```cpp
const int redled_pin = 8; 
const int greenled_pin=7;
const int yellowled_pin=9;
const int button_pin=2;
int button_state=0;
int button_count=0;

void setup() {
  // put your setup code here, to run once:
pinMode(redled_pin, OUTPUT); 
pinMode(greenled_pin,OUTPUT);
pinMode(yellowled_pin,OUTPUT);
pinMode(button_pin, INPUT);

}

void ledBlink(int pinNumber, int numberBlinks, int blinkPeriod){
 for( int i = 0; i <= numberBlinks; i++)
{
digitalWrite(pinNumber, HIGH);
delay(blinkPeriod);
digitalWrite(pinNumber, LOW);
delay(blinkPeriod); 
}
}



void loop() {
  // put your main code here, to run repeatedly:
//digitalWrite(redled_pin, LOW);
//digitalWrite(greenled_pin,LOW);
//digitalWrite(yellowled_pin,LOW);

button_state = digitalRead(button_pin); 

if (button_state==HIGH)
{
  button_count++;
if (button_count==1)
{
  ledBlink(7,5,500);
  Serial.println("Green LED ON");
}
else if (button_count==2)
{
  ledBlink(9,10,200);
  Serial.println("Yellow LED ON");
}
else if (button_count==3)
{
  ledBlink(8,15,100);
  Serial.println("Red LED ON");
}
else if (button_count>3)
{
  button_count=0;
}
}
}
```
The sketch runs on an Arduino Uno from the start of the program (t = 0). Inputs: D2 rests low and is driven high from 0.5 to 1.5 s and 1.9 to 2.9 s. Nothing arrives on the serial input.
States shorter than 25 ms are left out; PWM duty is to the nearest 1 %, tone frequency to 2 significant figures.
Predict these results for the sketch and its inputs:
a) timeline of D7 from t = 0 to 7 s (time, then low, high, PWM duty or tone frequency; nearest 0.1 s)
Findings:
0 s low; 0.5 s high; 1 s low; 1.5 s high; 2 s low; 2.5 s high; 3 s low; 3.5 s high; 4 s low; 4.5 s high; 5 s low; 5.5 s high; 6 s low
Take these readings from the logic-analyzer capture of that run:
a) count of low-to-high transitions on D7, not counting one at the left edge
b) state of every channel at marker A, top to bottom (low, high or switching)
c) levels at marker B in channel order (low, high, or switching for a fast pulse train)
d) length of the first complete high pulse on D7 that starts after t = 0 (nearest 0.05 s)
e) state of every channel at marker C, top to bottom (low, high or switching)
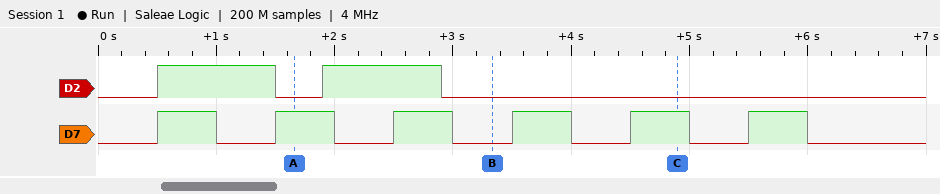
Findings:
6
D2 low, D7 high
D2 low, D7 low
0.50 s
D2 low, D7 high
